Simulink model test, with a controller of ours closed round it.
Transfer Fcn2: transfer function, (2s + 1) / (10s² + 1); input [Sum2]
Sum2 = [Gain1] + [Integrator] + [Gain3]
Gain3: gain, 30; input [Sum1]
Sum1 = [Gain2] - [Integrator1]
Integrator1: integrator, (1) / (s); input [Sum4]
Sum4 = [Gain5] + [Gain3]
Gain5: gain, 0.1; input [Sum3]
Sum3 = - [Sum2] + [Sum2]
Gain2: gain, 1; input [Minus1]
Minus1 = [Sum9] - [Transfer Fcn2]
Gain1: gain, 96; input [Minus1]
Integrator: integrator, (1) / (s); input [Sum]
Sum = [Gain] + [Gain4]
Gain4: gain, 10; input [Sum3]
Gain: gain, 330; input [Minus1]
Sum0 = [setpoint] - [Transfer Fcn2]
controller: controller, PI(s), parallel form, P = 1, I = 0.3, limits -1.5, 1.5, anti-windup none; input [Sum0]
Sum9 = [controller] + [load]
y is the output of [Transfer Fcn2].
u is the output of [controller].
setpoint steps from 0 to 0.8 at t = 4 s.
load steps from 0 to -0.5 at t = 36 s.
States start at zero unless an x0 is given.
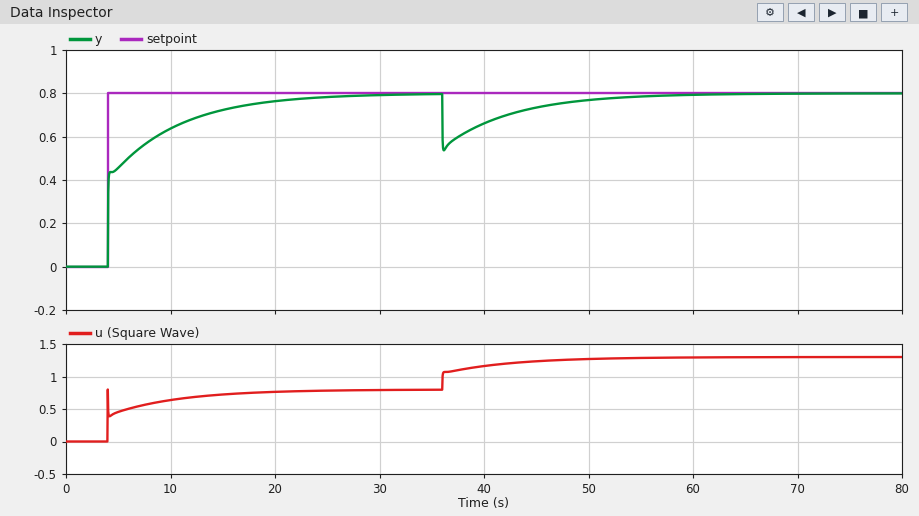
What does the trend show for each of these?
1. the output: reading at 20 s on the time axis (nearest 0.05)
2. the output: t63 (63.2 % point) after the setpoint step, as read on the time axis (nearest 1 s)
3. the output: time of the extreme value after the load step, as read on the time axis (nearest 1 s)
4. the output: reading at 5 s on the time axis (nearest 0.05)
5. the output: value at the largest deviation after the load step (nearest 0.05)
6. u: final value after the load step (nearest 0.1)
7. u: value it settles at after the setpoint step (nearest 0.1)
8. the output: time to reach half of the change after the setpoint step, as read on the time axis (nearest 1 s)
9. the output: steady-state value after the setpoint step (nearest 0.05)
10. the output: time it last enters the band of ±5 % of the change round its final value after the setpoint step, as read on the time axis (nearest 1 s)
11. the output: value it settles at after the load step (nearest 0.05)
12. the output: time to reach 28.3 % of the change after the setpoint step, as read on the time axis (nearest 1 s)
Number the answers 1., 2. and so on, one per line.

1. 0.75
2. 6 s
3. 36 s
4. 0.45
5. 0.55
6. 1.3
7. 0.8
8. 4 s
9. 0.80
10. 19 s
11. 0.80
12. 4 s
